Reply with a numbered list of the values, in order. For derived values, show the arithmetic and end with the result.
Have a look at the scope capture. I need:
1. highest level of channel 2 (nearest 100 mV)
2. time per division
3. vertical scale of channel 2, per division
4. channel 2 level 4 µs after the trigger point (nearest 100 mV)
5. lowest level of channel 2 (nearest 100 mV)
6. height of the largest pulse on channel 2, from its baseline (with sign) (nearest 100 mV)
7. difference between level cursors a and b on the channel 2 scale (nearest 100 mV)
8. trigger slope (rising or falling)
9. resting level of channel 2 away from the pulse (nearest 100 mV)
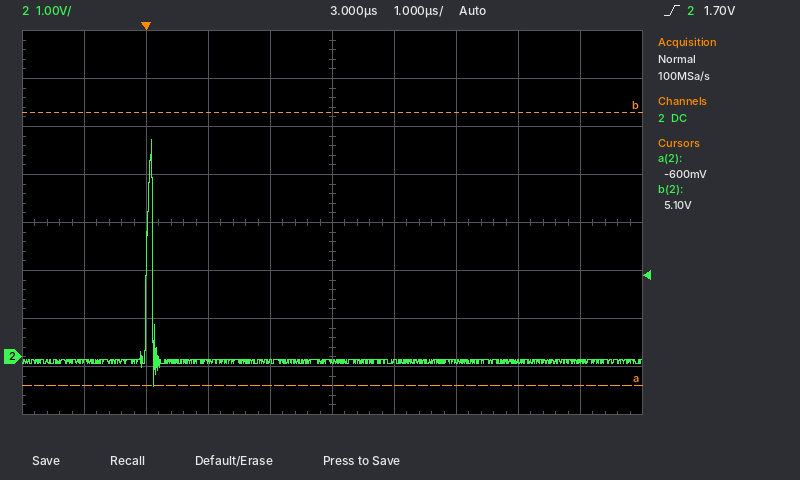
1. 4.5 V
2. 1 µs
3. 1 V
4. -100 mV
5. -600 mV
6. 4.5 V − (-100 mV) = +4.6 V
7. 5.7 V
8. rising
9. -100 mV
